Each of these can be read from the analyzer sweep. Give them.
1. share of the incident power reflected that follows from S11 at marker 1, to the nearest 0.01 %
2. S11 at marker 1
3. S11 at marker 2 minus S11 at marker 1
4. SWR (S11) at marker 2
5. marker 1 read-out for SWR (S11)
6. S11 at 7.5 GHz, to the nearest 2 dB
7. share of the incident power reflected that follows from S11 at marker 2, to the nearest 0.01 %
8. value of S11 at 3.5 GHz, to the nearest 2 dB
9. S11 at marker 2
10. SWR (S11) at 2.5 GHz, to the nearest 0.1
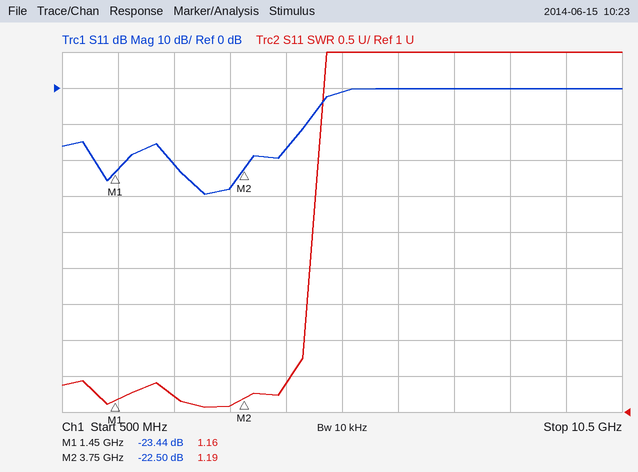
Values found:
0.45 %
-23.44 dB
0.94 dB
1.19
1.16
0 dB
0.56 %
-28 dB
-22.50 dB
1.2
